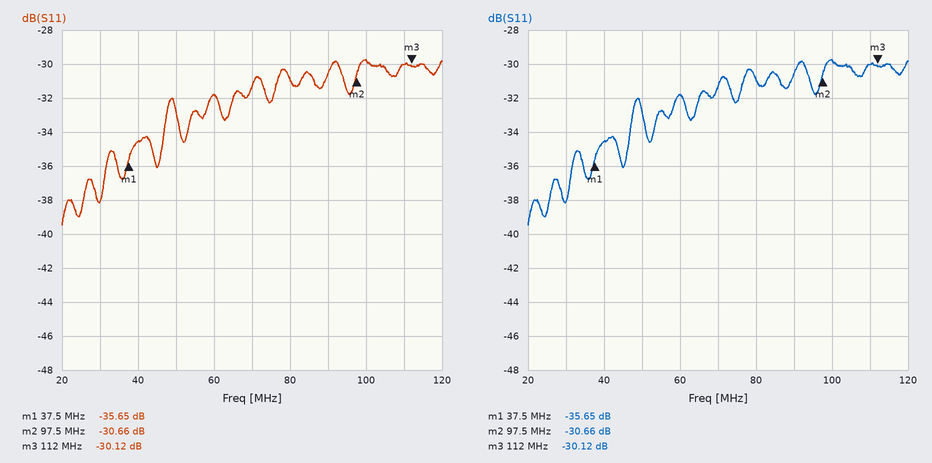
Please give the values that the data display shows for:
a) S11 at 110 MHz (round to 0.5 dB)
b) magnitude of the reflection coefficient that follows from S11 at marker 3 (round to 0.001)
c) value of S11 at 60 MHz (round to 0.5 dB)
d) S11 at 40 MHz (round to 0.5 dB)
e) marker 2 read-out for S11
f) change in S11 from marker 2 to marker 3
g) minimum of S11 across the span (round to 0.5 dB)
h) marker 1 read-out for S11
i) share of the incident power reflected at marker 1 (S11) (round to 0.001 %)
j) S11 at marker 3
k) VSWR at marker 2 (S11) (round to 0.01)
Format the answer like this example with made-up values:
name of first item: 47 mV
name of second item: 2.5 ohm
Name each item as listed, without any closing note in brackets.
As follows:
S11 at 110 MHz: -30.0 dB
magnitude of the reflection coefficient that follows from S11 at marker 3: 0.031
value of S11 at 60 MHz: -32.0 dB
S11 at 40 MHz: -34.5 dB
marker 2 read-out for S11: -30.66 dB
change in S11 from marker 2 to marker 3: 0.54 dB
minimum of S11 across the span: -39.5 dB
marker 1 read-out for S11: -35.65 dB
share of the incident power reflected at marker 1 (S11): 0.027 %
S11 at marker 3: -30.12 dB
VSWR at marker 2 (S11): 1.06
